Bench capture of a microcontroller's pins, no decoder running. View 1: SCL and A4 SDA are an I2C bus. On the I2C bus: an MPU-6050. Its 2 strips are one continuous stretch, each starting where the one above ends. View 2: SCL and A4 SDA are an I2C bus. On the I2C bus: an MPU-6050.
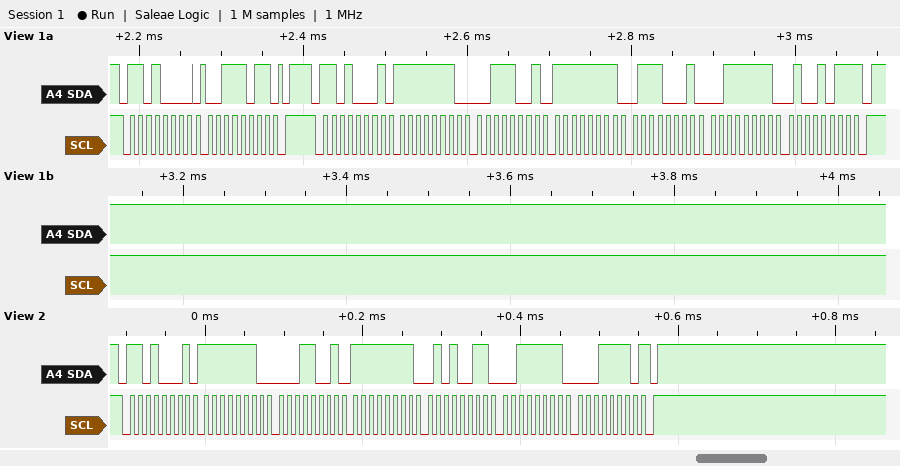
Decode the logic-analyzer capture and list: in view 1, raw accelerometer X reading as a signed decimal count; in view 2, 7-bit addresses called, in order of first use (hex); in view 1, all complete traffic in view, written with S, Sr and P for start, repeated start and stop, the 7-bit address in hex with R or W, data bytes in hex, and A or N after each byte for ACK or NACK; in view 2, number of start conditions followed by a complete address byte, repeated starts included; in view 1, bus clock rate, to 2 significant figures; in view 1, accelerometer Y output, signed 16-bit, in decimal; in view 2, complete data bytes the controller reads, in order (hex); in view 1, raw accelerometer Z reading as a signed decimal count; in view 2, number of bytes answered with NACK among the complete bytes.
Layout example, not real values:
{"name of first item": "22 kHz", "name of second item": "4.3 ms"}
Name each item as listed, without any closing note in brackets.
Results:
{"in view 1, raw accelerometer X reading as a signed decimal count": "-455", "in view 2, 7-bit addresses called, in order of first use": "0x68", "in view 1, all complete traffic in view, written with S, Sr and P for start, repeated start and stop, the 7-bit address in hex with R or W, data bytes in hex, and A or N after each byte for ACK or NACK": "S 68W A 3B A P S 68R A FE A 39 A FF A 71 A 3F A 4B N P", "in view 2, number of start conditions followed by a complete address byte, repeated starts included": "1", "in view 1, bus clock rate, to 2 significant figures": "100 kHz", "in view 1, accelerometer Y output, signed 16-bit, in decimal": "-143", "in view 2, complete data bytes the controller reads, in order": "FE 19 FF 53 3F 1E", "in view 1, raw accelerometer Z reading as a signed decimal count": "16203", "in view 2, number of bytes answered with NACK among the complete bytes": "1"}
